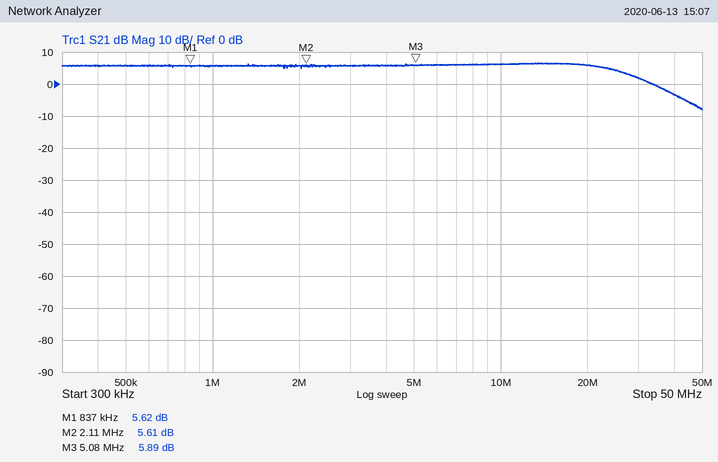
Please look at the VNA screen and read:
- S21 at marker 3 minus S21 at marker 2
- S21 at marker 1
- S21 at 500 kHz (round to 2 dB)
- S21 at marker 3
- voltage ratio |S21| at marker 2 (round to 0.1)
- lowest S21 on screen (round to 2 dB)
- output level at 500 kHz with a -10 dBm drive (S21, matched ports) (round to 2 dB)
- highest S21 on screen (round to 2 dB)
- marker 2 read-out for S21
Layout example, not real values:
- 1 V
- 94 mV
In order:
- 0.28 dB
- 5.62 dB
- 6 dB
- 5.89 dB
- 1.9
- -8 dB
- -4 dBm
- 6 dB
- 5.61 dB
